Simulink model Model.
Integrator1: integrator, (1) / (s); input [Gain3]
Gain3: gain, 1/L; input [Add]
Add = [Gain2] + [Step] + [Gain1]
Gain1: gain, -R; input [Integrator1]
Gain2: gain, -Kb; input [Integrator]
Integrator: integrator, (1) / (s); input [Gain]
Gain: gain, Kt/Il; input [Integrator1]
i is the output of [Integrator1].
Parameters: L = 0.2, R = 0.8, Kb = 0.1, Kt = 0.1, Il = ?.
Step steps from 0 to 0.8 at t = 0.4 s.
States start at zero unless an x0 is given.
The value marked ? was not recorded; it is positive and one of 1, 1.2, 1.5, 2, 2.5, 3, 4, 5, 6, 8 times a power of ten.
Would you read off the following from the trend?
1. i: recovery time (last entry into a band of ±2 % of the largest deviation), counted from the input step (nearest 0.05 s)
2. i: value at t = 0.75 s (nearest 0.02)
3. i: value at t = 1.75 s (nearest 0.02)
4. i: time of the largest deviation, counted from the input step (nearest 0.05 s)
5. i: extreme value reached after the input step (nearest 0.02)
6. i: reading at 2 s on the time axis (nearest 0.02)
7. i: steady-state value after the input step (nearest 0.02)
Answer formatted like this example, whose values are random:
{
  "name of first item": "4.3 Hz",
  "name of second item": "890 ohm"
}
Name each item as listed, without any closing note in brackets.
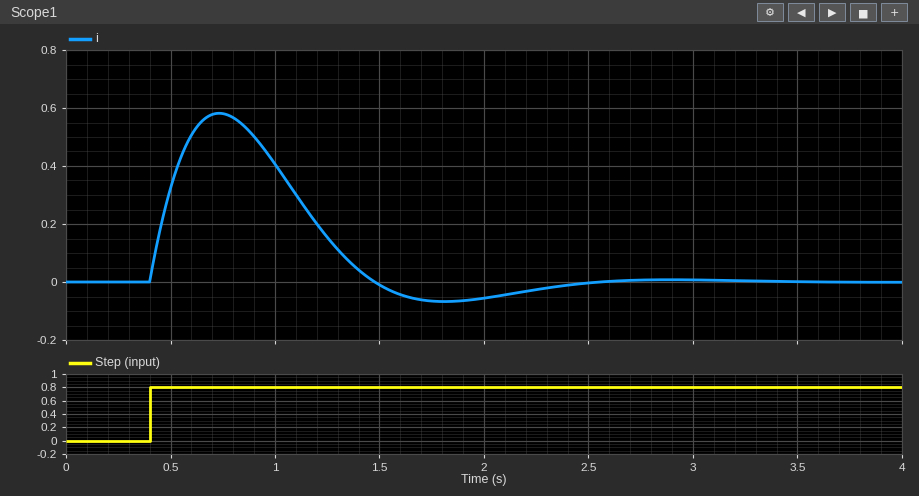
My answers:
{
  "i: recovery time (last entry into a band of ±2 % of the largest deviation), counted from the input step": "2.00 s",
  "i: value at t = 0.75 s": "0.58",
  "i: value at t = 1.75 s": "-0.06",
  "i: time of the largest deviation, counted from the input step": "0.35 s",
  "i: extreme value reached after the input step": "0.58",
  "i: reading at 2 s on the time axis": "-0.06",
  "i: steady-state value after the input step": "0.00"
}
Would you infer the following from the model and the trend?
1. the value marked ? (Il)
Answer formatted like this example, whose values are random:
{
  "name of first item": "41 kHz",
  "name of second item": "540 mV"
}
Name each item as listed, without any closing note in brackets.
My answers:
{
  "the value marked ?": "0.004"
}
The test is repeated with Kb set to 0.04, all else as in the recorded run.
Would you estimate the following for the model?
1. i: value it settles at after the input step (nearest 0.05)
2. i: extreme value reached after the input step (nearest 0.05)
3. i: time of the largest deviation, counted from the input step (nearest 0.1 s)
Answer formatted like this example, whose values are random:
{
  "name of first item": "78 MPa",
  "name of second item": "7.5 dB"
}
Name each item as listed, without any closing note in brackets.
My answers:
{
  "i: value it settles at after the input step": "0.00",
  "i: extreme value reached after the input step": "0.70",
  "i: time of the largest deviation, counted from the input step": "0.5 s"
}
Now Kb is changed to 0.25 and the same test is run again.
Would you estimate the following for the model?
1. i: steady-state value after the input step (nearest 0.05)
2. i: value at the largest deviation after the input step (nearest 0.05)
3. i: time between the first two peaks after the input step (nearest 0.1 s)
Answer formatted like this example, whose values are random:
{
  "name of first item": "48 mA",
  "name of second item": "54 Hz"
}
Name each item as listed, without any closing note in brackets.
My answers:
{
  "i: steady-state value after the input step": "0.00",
  "i: value at the largest deviation after the input step": "0.45",
  "i: time between the first two peaks after the input step": "1.2 s"
}
